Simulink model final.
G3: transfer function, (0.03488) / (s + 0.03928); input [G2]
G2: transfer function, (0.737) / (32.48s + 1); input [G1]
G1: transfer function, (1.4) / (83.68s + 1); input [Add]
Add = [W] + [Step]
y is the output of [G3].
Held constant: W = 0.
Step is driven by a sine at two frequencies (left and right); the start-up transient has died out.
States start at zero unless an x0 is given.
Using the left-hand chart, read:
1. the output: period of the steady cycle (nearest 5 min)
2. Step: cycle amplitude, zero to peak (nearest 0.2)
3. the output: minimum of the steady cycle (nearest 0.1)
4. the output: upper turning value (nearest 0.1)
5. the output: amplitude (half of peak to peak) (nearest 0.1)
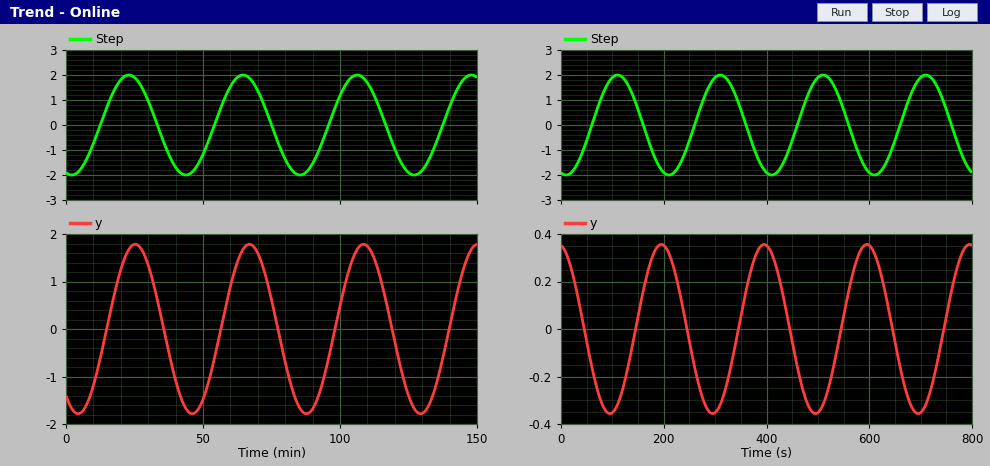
40 min
2.0
-1.8
1.8
1.8
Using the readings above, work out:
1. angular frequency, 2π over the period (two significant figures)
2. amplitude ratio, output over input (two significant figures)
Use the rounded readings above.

0.16 rad/min
0.90
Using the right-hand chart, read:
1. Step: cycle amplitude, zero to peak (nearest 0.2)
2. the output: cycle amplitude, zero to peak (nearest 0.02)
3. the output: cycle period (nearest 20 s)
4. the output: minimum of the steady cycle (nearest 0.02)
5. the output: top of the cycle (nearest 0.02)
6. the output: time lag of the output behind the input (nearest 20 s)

2.0
0.36
200 s
-0.36
0.36
80 s
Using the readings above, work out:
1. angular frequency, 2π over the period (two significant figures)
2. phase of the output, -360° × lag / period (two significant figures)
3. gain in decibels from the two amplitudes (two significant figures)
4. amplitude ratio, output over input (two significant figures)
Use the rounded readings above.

0.031 rad/s
-140°
-15 dB
0.18
